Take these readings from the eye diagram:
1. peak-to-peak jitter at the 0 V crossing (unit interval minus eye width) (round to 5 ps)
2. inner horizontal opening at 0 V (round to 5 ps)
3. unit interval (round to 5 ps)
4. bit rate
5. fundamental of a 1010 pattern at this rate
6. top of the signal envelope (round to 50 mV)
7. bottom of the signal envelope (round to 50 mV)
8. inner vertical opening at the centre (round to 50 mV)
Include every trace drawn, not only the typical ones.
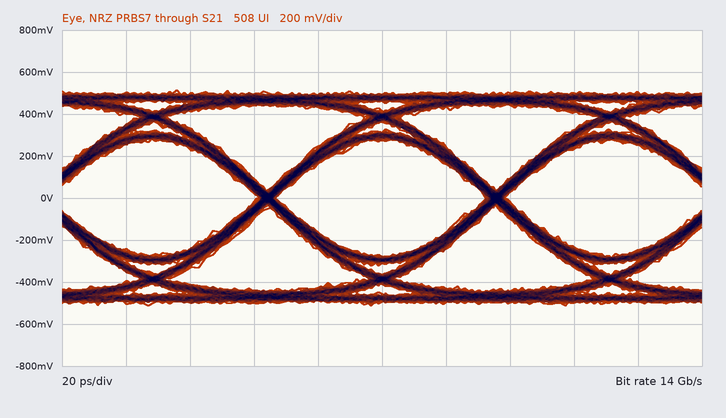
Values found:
5 ps
65 ps
70 ps
14 Gb/s
7 GHz
500 mV
-500 mV
550 mV
